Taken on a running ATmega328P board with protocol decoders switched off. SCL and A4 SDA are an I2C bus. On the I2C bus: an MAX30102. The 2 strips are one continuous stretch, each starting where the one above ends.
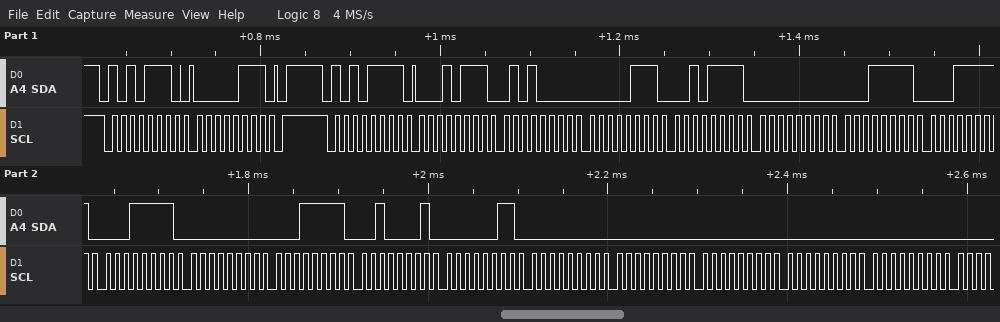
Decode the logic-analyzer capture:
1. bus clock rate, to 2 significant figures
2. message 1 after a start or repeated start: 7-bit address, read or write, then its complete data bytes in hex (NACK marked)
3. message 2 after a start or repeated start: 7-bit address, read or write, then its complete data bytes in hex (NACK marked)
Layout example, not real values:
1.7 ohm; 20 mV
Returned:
100 kHz; 0x57 write: 07; 0x57 read: 17 50 07 2F 00 1F 1F 1F 00 1F 21 03 00 00 00 00 00
